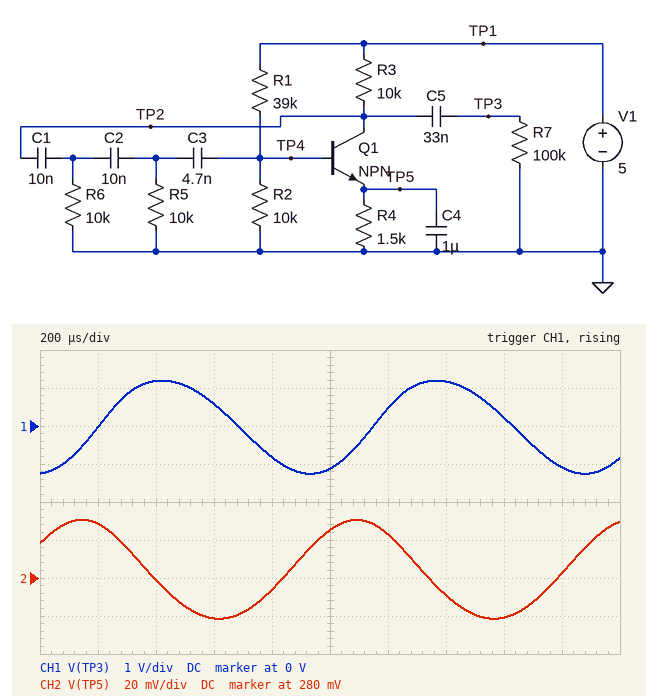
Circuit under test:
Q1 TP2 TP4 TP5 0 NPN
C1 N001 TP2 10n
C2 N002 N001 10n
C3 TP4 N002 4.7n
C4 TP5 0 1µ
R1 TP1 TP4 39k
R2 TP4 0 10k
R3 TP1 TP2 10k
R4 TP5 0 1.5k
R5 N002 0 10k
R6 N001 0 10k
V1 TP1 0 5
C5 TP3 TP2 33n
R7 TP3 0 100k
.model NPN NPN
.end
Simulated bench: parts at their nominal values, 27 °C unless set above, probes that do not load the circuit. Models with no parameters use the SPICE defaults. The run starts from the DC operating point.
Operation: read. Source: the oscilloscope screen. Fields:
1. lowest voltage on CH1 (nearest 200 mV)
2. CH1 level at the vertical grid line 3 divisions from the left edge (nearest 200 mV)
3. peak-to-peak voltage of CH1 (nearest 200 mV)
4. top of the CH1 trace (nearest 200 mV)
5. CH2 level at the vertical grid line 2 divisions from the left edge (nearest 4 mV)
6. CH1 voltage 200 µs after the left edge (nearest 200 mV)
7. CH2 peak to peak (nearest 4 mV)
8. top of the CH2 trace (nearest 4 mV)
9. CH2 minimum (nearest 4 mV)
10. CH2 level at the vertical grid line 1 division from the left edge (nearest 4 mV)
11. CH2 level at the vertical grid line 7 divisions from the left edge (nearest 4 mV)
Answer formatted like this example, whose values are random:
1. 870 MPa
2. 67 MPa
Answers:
1. -1.2 V
2. 600 mV
3. 2.4 V
4. 1.2 V
5. 280 mV
6. 0 V
7. 52 mV
8. 312 mV
9. 260 mV
10. 308 mV
11. 272 mV
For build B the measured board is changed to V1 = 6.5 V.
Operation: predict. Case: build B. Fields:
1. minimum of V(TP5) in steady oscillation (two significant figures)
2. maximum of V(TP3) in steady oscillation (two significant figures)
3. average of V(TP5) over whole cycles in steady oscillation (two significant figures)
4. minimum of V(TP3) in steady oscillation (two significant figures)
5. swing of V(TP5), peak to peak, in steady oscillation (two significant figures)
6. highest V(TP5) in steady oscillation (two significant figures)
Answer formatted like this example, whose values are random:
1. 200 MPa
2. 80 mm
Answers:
1. 490 mV
2. 2.3 V
3. 540 mV
4. -2.4 V
5. 99 mV
6. 590 mV
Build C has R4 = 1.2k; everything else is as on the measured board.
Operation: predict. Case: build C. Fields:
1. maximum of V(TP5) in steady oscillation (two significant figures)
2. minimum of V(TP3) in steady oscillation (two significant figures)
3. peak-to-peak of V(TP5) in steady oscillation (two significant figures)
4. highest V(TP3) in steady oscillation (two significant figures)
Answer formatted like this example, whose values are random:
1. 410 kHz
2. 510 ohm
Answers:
1. 320 mV
2. -1.7 V
3. 72 mV
4. 1.6 V
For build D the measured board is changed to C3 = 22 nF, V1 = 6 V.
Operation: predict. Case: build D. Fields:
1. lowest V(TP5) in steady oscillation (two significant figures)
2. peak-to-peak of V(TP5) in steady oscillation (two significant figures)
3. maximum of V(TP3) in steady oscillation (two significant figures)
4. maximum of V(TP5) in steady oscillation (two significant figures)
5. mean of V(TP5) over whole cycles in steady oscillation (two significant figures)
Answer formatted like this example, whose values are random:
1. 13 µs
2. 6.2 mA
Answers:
1. 390 mV
2. 140 mV
3. 2.3 V
4. 530 mV
5. 460 mV
